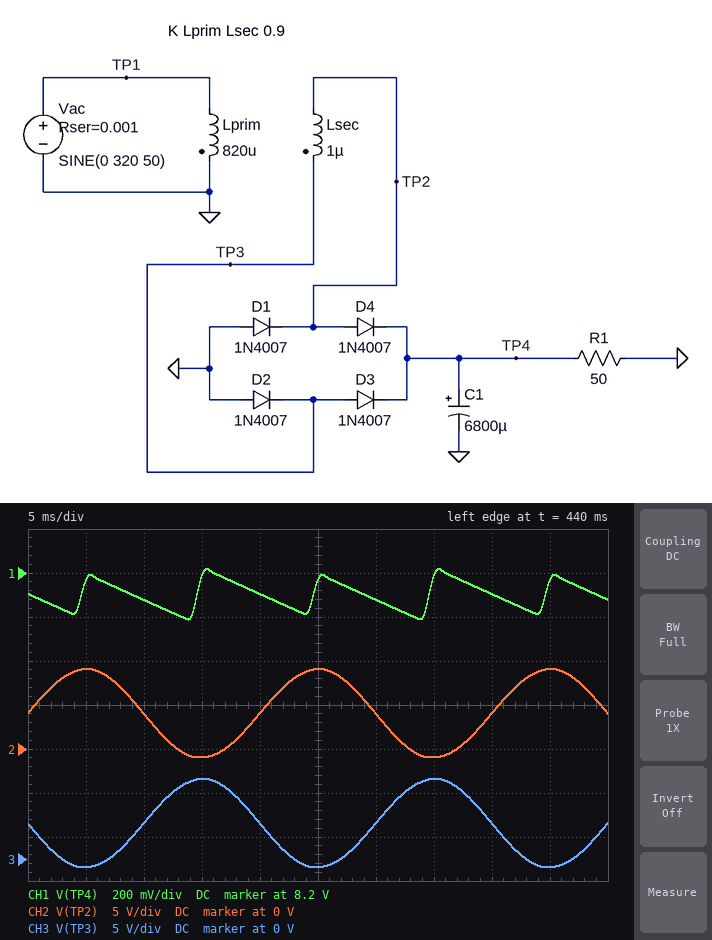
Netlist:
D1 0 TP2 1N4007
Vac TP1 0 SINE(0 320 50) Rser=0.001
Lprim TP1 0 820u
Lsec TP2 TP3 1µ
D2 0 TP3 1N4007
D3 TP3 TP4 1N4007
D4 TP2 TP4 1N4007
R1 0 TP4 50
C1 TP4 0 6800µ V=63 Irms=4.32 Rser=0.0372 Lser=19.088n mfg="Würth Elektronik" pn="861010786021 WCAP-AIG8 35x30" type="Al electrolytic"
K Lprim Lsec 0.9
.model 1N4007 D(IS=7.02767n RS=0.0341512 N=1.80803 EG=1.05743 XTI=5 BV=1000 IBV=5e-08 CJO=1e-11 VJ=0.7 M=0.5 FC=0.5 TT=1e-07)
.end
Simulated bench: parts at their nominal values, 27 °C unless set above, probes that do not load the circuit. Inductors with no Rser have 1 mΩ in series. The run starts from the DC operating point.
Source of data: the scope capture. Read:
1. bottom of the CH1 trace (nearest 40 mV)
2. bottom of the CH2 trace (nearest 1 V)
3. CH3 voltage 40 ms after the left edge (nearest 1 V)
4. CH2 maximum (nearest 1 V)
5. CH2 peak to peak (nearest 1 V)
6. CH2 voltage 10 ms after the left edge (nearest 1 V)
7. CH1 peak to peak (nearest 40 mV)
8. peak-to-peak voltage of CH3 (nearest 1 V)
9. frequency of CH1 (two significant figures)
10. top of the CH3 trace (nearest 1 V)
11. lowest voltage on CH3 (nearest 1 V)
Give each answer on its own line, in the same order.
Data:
8.00 V
-1 V
4 V
9 V
10 V
4 V
240 mV
10 V
100 Hz
9 V
-1 V
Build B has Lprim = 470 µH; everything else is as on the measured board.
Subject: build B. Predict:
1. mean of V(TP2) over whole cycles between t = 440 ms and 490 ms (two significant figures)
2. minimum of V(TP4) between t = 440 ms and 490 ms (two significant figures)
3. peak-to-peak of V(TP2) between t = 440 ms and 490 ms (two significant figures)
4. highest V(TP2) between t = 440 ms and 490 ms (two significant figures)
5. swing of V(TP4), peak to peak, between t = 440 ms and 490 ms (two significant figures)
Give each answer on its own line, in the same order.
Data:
5.6 V
11 V
13 V
12 V
320 mV
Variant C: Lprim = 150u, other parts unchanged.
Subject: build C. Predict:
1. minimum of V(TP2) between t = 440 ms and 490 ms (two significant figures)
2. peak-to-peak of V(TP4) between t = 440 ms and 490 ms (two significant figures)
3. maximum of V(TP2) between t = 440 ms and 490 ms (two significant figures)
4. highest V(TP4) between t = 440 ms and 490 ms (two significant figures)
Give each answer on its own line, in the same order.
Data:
-1.1 V
560 mV
22 V
21 V
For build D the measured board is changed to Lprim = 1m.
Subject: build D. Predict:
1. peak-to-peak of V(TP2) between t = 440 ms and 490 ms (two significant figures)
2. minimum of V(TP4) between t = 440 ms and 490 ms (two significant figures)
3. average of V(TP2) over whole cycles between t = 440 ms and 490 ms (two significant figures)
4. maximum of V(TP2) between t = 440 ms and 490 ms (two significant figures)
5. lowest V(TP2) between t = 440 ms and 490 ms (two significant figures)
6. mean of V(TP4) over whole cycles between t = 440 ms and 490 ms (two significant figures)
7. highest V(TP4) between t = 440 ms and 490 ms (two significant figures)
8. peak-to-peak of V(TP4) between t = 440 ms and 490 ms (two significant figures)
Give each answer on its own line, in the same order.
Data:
9.1 V
7.1 V
3.6 V
8.2 V
-940 mV
7.2 V
7.3 V
200 mV
